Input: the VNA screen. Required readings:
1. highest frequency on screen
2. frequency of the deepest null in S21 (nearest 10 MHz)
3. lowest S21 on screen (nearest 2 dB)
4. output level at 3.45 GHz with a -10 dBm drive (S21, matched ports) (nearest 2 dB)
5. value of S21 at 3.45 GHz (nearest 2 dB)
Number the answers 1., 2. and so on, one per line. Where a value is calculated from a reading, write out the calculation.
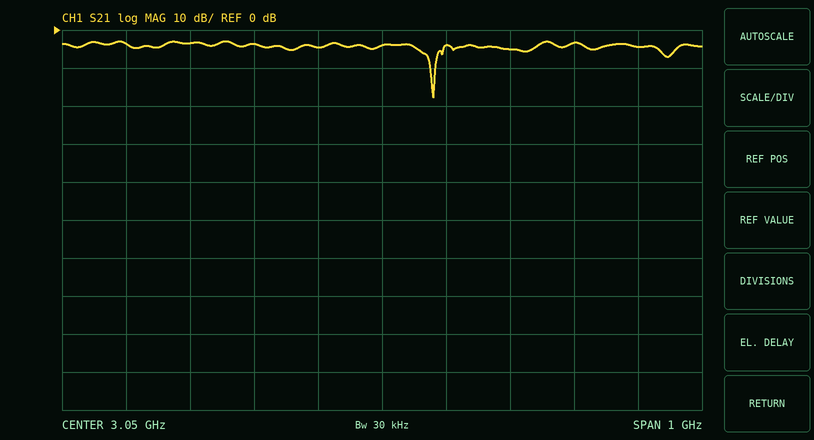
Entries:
1. 3.55 GHz
2. 3.13 GHz
3. -18 dB
4. -10 dBm + (-4 dB) = -14 dBm
5. -4 dB
